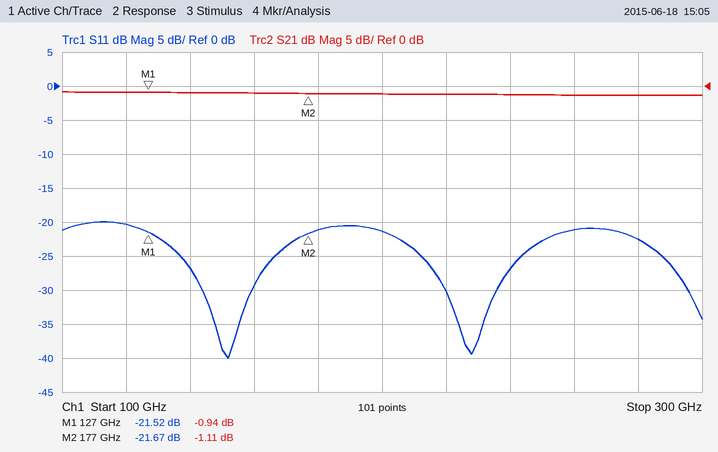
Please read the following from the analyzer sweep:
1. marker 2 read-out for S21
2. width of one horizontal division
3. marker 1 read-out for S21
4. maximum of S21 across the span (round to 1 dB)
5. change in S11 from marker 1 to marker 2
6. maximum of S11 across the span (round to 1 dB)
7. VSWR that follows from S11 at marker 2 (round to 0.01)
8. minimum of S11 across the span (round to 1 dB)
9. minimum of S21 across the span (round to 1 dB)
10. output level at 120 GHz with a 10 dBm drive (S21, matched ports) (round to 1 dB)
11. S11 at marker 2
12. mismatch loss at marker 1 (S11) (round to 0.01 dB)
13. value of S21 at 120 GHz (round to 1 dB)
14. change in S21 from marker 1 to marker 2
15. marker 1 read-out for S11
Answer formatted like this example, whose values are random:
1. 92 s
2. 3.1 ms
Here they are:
1. -1.11 dB
2. 20 GHz
3. -0.94 dB
4. -1 dB
5. -0.15 dB
6. -20 dB
7. 1.18
8. -40 dB
9. -1 dB
10. 9 dBm
11. -21.67 dB
12. 0.03 dB
13. -1 dB
14. -0.17 dB
15. -21.52 dB
